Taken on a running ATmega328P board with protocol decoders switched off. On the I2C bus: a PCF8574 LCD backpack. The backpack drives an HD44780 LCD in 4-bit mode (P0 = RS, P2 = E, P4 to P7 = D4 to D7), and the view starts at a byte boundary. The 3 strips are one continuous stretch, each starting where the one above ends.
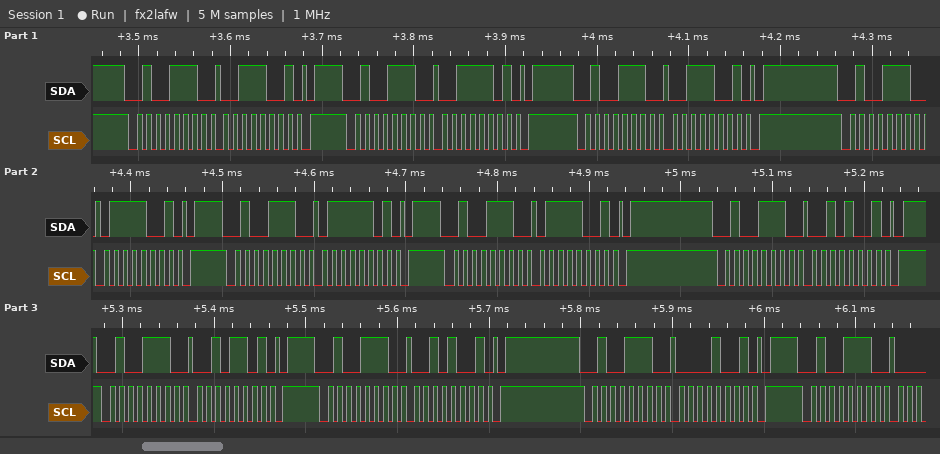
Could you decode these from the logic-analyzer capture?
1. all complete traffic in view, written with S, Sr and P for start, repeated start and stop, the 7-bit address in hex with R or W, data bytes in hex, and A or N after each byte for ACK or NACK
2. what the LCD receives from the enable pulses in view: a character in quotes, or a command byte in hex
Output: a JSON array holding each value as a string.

["S 27W A 39 A P S 27W A 3D A P S 27W A 39 A P S 27W A 79 A P S 27W A 7D A P S 27W A 79 A P S 27W A 29 A P S 27W A 2D A P S 27W A 29 A P S 27W A 09 A P S 27W A", "'7'"]
